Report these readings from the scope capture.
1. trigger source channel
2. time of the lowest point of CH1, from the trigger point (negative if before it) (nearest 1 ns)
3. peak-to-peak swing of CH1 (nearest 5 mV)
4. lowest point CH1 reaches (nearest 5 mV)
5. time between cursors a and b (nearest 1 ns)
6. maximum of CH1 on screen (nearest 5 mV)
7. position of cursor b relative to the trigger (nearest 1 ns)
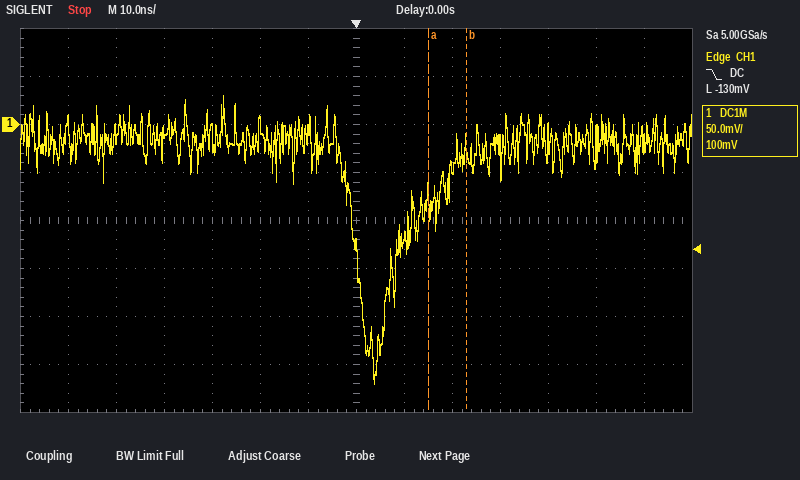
CH1
+4 ns
300 mV
-270 mV
8 ns
30 mV
+23 ns
